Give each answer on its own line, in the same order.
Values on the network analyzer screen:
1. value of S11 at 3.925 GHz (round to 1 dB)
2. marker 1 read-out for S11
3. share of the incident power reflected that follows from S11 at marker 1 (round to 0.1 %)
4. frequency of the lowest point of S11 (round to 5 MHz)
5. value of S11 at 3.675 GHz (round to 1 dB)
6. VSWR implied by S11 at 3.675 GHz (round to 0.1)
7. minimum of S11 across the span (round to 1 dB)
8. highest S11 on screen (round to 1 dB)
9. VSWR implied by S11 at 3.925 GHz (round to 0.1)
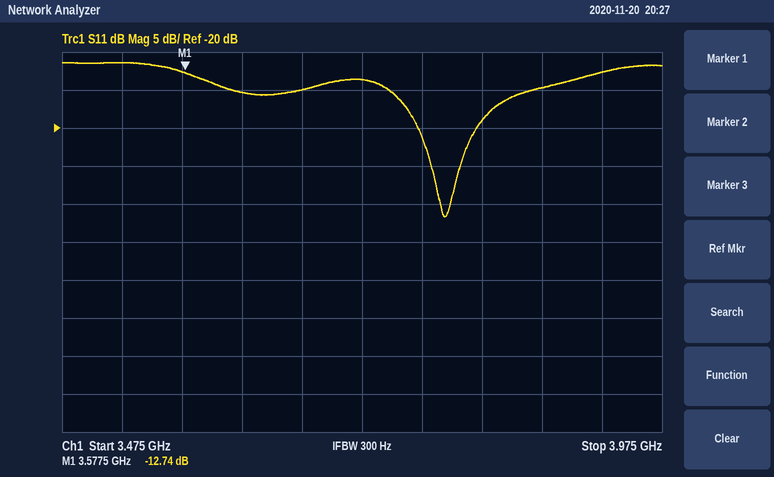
-13 dB
-12.74 dB
5.3 %
3.795 GHz
-15 dB
1.4
-32 dB
-11 dB
1.6
